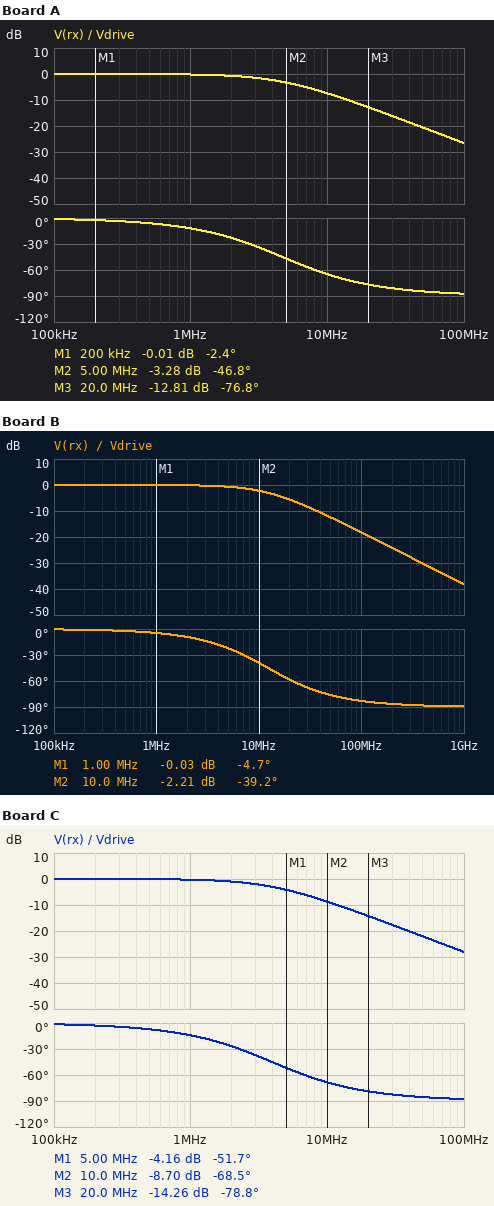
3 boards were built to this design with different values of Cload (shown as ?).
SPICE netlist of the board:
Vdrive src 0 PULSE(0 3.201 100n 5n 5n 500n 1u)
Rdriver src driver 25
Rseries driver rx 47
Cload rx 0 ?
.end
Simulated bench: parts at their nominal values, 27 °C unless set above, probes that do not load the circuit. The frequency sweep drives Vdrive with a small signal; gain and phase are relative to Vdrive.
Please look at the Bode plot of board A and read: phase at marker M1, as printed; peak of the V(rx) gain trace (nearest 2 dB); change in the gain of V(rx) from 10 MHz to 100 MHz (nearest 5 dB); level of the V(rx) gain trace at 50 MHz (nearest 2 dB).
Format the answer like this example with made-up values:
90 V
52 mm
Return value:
-2.4 deg
0 dB
-20 dB
-20 dB
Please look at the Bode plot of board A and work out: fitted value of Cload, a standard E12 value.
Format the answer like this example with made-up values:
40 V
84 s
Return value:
470 pF
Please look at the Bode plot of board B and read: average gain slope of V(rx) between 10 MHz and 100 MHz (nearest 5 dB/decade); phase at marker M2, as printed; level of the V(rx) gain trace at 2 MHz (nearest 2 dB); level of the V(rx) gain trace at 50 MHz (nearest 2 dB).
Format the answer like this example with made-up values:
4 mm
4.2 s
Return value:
-15 dB/decade
-39.2 deg
0 dB
-12 dB
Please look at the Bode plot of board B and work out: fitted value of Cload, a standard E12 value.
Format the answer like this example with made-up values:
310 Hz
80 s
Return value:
180 pF
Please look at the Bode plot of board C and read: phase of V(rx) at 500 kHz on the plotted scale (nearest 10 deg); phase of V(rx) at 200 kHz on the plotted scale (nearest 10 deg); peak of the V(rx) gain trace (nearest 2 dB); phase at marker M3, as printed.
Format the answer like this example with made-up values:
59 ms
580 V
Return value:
-10 deg
0 deg
0 dB
-78.8 deg
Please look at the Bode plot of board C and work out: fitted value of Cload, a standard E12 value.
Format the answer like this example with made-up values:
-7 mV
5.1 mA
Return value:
560 pF
